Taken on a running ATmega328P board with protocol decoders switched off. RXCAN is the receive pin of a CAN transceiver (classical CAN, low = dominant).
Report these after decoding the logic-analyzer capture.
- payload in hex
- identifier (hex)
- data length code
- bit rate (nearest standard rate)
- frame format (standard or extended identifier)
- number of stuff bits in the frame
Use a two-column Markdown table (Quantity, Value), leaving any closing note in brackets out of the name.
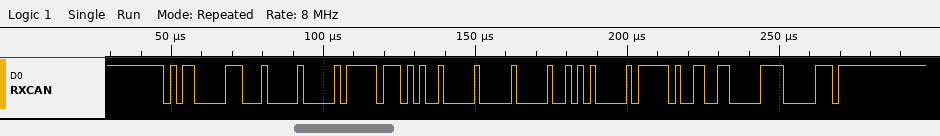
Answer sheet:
| Quantity | Value |
|---|---|
| payload in hex | 00 FF 52 00 00 A8 1F 99 |
| identifier | 0x583 |
| data length code | 8 |
| bit rate | 500 kbit/s |
| frame format | standard |
| number of stuff bits in the frame | 11 |
